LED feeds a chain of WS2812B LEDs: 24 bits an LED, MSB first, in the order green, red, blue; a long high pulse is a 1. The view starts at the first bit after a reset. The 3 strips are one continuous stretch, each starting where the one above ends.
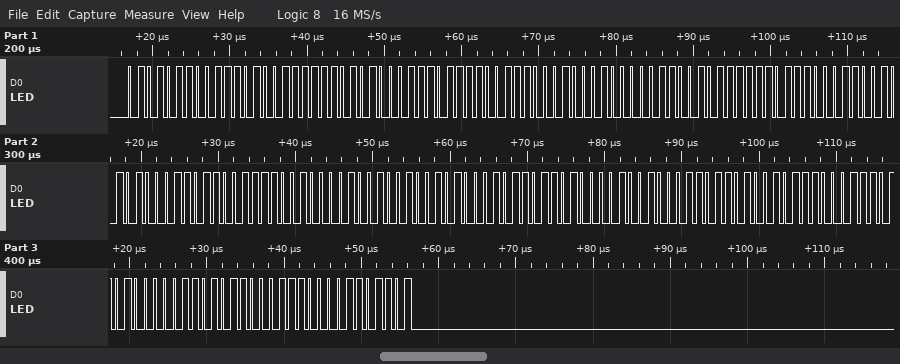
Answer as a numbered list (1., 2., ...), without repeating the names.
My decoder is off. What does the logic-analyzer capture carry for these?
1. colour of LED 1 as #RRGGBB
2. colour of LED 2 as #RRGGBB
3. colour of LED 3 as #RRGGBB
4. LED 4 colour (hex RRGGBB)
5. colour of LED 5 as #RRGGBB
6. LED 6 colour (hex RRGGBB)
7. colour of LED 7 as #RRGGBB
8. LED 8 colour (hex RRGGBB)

1. #7456FD
2. #7947C4
3. #9741EE
4. #A33267
5. #929051
6. #096D1B
7. #8E4BA0
8. #38D66D
